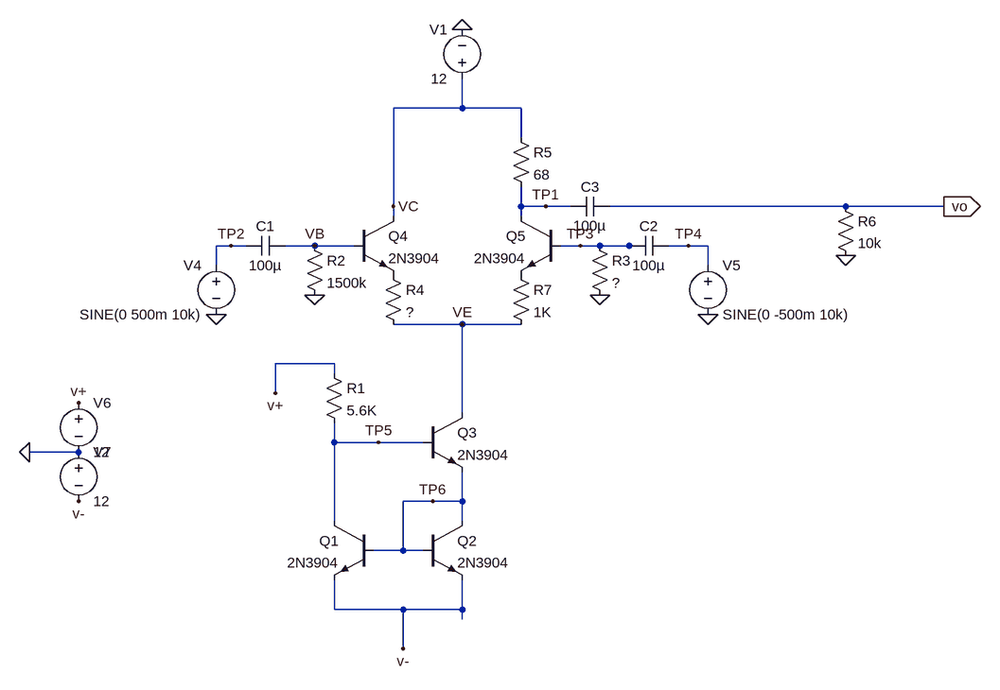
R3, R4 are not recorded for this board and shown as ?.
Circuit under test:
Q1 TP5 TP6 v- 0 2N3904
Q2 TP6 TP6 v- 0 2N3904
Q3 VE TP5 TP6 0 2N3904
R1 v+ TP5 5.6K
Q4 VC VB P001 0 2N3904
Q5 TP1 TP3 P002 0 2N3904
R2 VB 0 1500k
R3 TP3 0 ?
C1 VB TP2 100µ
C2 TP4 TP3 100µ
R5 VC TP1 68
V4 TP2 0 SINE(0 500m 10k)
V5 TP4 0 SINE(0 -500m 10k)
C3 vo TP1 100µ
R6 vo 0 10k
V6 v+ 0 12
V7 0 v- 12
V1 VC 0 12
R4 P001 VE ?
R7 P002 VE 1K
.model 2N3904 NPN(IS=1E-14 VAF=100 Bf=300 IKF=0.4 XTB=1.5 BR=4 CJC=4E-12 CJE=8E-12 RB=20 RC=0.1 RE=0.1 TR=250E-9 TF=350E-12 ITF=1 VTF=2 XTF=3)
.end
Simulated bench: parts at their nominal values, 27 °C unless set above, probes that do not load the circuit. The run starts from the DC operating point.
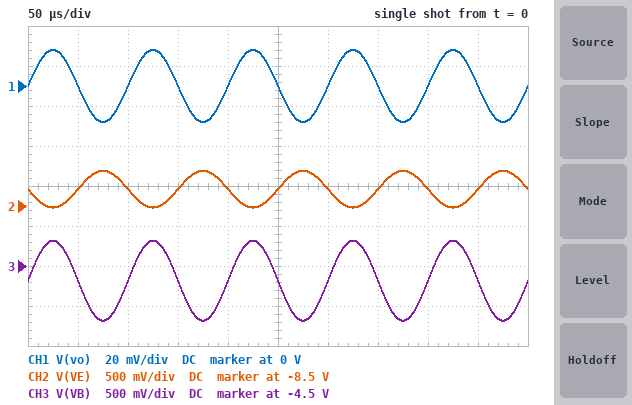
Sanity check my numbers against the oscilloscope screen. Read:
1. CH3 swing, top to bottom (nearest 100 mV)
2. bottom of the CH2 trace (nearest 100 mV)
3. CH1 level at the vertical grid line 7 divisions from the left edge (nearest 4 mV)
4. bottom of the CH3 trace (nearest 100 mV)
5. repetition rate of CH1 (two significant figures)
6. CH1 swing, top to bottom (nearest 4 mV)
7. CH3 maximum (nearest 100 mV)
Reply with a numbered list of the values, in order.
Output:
1. 1.0 V
2. -8.5 V
3. 0 V
4. -5.2 V
5. 10 kHz
6. 36 mV
7. -4.2 V
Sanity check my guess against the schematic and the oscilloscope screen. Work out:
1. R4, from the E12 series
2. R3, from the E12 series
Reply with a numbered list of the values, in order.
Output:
1. 2.7 kΩ
2. 560 kΩ
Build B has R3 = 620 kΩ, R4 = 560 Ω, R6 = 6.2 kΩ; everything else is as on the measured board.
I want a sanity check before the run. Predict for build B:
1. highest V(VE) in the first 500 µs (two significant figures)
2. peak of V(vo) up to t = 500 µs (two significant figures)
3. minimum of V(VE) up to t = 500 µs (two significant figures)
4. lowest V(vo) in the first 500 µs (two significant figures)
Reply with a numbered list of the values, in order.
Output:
1. -7.6 V
2. 42 mV
3. -7.9 V
4. -42 mV
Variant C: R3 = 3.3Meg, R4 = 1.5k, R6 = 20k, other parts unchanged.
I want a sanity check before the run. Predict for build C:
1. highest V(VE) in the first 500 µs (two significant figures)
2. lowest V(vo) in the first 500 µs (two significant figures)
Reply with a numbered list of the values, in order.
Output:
1. -11 V
2. -33 mV
